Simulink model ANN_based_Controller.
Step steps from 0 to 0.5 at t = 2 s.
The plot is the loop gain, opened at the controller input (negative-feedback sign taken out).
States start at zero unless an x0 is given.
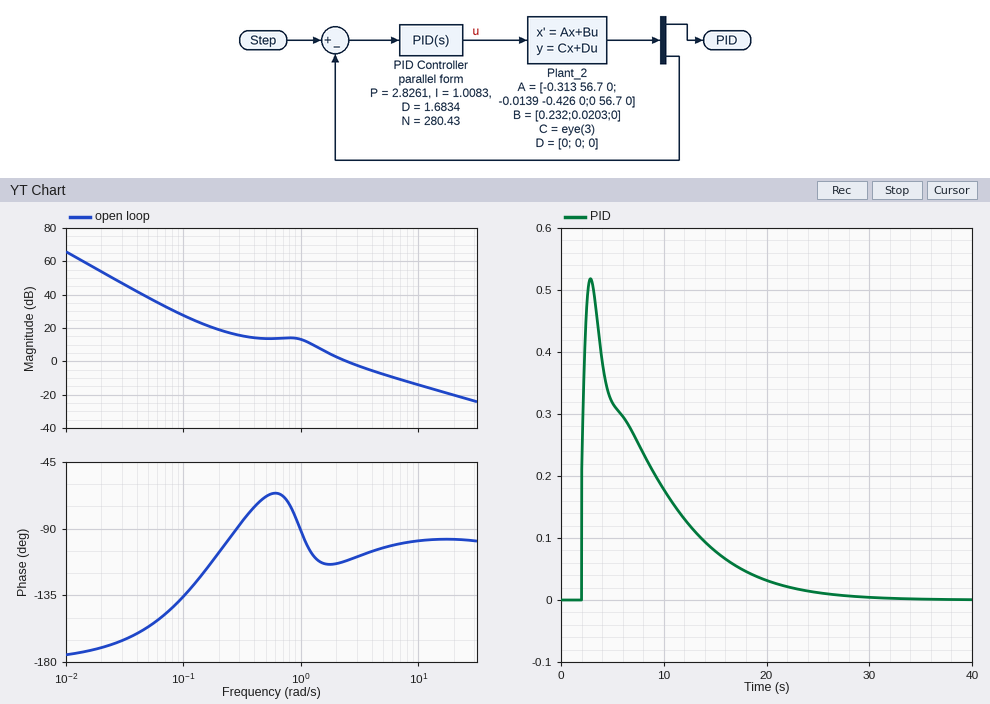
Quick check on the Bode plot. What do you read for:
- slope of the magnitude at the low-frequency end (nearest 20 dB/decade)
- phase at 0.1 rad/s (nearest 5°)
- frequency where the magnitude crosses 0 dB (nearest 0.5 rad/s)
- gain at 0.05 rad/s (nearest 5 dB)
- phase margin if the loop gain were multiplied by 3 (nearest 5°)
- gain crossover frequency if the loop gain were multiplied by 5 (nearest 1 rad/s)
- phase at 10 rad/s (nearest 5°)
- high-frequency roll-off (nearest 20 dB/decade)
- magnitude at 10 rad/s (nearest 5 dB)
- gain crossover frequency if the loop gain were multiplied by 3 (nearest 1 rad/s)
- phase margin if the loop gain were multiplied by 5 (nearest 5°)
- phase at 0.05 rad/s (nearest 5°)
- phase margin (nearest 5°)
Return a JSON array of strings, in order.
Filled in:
["-40 dB/decade", "-135°", "2.5 rad/s", "40 dB", "80°", "10 rad/s", "-100°", "-20 dB/decade", "-15 dB", "6 rad/s", "80°", "-155°", "70°"]
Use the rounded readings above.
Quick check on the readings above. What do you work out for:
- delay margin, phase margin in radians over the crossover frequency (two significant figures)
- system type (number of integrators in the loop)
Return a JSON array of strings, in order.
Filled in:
["0.49 s", "2"]
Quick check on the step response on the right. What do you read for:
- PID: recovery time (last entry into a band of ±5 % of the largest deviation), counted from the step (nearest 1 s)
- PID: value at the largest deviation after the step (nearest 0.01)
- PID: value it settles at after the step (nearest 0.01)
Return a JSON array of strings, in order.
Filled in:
["19 s", "0.52", "0.00"]
